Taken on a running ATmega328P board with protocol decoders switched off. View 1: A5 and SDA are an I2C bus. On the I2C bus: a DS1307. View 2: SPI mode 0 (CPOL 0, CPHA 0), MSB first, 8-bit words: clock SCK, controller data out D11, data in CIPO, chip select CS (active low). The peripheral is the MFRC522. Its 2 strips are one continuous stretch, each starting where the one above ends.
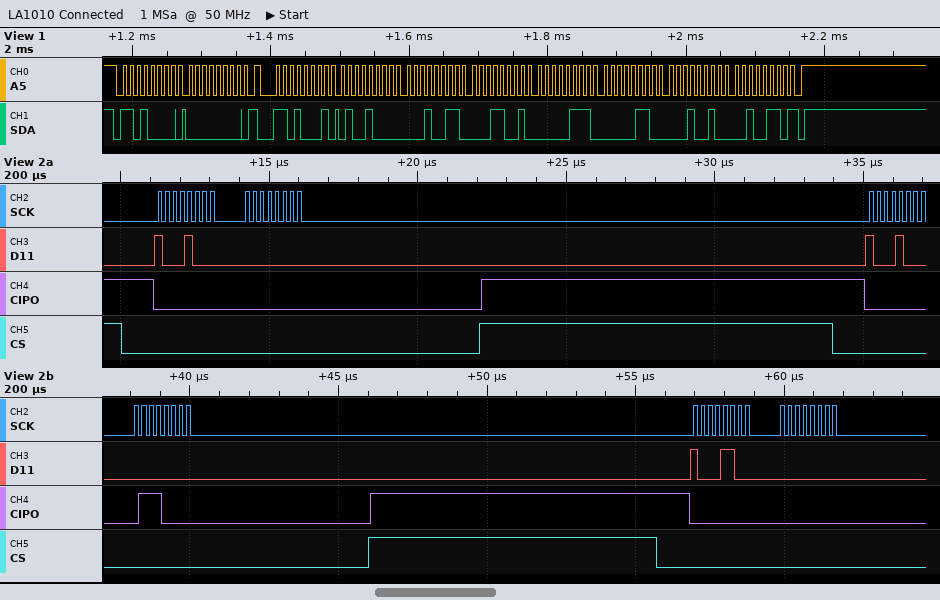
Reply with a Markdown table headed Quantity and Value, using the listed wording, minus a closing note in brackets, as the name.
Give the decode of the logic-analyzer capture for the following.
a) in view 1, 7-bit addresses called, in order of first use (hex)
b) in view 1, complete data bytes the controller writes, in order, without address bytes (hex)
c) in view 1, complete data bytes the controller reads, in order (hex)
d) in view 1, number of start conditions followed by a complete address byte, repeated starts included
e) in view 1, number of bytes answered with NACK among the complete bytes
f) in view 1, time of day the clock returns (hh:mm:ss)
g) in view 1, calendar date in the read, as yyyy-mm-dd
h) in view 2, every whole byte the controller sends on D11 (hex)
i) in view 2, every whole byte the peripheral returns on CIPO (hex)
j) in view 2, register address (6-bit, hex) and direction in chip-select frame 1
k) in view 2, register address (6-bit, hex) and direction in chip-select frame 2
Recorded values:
| Quantity | Value |
|---|---|
| in view 1, 7-bit addresses called, in order of first use | 0x68 |
| in view 1, complete data bytes the controller writes, in order, without address bytes | 00 |
| in view 1, complete data bytes the controller reads, in order | 48 13 19 07 06 12 26 |
| in view 1, number of start conditions followed by a complete address byte, repeated starts included | 2 |
| in view 1, number of bytes answered with NACK among the complete bytes | 1 |
| in view 1, time of day the clock returns | 19:13:48 |
| in view 1, calendar date in the read, as yyyy-mm-dd | 2026-12-06 |
| in view 2, every whole byte the controller sends on D11 | 88 00 88 00 8C 00 |
| in view 2, every whole byte the peripheral returns on CIPO | 00 00 00 70 00 00 |
| in view 2, register address (6-bit, hex) and direction in chip-select frame 1 | 0x04 read |
| in view 2, register address (6-bit, hex) and direction in chip-select frame 2 | 0x04 read |
